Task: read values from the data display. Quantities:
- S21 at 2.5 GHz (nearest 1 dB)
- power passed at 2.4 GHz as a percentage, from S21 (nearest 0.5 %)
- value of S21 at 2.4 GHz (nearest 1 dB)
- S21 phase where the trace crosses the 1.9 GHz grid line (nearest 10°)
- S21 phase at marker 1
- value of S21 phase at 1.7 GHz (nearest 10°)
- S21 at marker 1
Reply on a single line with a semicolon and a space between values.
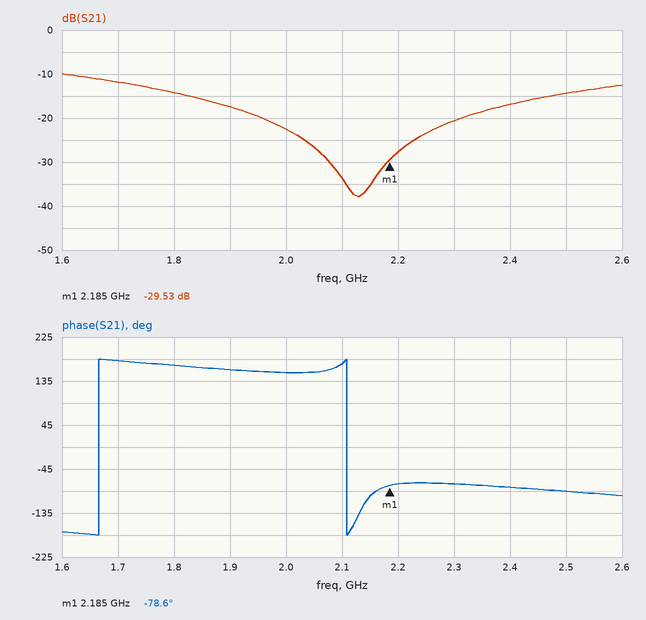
-14 dB; 2.0 %; -17 dB; 160°; -78.6°; 180°; -29.53 dB
